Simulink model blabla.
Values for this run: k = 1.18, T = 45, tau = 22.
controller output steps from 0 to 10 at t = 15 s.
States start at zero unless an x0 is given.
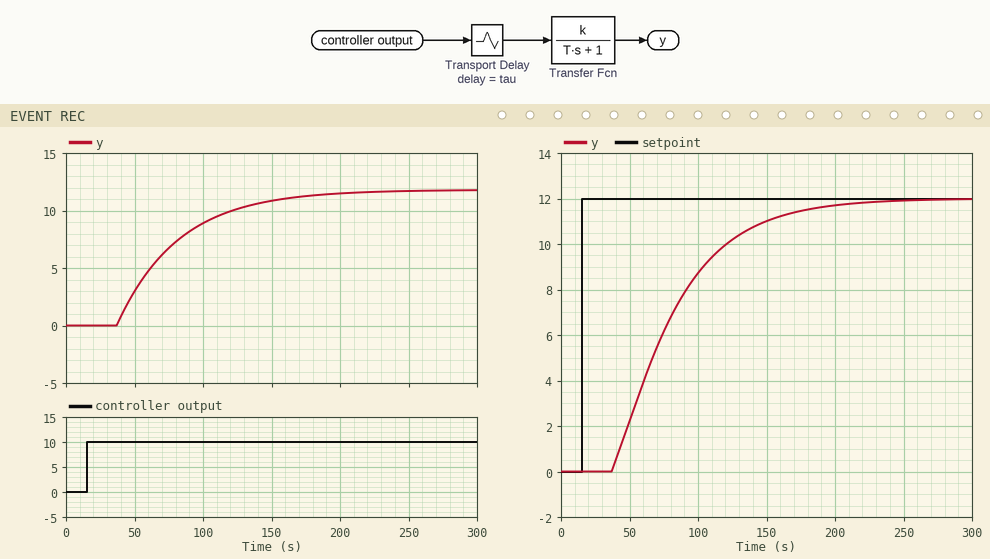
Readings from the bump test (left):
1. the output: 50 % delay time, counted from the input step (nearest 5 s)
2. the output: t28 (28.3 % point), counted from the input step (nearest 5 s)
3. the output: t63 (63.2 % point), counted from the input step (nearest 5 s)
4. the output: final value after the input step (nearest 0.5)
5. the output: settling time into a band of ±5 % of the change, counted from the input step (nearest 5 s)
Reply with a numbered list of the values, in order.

1. 55 s
2. 35 s
3. 65 s
4. 12.0
5. 155 s
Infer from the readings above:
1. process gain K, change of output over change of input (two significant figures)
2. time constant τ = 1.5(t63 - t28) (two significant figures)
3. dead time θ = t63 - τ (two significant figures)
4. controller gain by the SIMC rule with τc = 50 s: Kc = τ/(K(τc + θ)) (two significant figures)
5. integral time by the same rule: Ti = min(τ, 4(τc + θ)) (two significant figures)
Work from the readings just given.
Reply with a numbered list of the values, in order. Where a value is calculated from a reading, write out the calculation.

1. (12 - 0) / 10 = 1.2
2. 1.5 × (65 - 35) = 45 s
3. 65 - 45 = 20 s
4. 45 / (1.2 × (50 + 20)) = 0.54
5. min(45, 4 × (50 + 20)) = 45 s
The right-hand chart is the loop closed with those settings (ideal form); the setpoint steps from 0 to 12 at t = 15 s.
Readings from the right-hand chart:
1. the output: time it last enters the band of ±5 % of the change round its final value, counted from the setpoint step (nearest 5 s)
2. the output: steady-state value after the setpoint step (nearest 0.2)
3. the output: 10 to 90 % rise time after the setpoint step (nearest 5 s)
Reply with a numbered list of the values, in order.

1. 155 s
2. 12.0
3. 100 s
